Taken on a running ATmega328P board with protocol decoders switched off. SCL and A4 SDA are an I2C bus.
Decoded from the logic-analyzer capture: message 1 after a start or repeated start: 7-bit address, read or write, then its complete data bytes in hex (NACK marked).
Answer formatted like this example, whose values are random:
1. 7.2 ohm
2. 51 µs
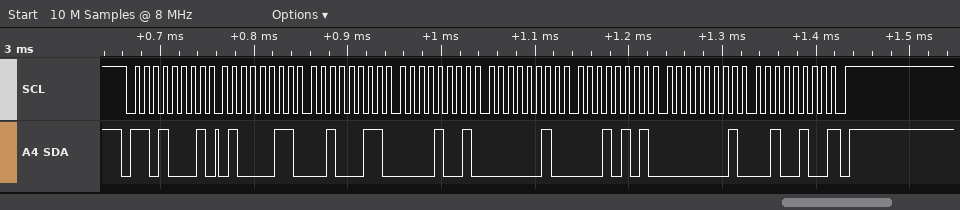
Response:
1. 0x68 read: 43 23 09 02 15 01 24 NACK
